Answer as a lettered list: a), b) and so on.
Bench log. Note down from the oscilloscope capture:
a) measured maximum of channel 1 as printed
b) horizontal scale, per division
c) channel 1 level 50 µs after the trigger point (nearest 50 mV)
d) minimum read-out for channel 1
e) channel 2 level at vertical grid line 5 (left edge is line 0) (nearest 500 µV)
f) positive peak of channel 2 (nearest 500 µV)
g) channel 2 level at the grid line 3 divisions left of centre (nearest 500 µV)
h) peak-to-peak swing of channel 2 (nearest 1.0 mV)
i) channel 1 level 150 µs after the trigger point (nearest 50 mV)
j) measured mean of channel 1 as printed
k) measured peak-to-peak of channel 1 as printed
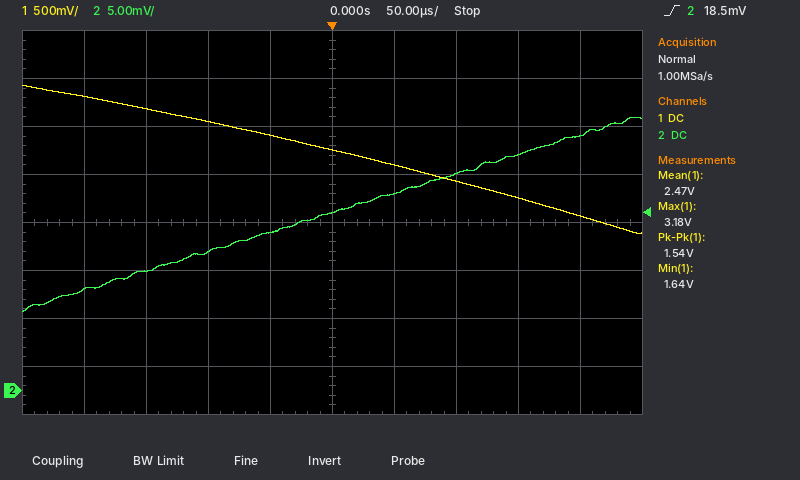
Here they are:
a) 3.18 V
b) 50 µs
c) 2.35 V
d) 1.64 V
e) 18.5 mV
f) 28.5 mV
g) 12.5 mV
h) 20.0 mV
i) 2.00 V
j) 2.47 V
k) 1.54 V
